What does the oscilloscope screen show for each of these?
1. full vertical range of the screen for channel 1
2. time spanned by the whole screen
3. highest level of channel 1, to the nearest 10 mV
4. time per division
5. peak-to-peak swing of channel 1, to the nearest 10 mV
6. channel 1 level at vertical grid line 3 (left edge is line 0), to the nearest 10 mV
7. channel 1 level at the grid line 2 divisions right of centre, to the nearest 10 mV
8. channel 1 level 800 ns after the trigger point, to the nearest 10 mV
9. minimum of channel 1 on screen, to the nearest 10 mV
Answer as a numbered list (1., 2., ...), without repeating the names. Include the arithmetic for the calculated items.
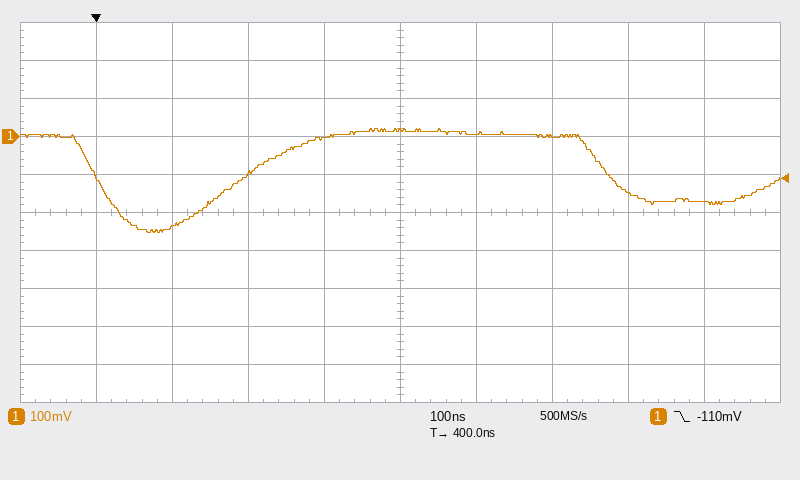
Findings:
1. 1 V
2. 1 µs
3. 20 mV
4. 100 ns
5. 20 mV − (-250 mV) = 270 mV
6. -100 mV
7. 0 mV
8. -170 mV
9. -250 mV
